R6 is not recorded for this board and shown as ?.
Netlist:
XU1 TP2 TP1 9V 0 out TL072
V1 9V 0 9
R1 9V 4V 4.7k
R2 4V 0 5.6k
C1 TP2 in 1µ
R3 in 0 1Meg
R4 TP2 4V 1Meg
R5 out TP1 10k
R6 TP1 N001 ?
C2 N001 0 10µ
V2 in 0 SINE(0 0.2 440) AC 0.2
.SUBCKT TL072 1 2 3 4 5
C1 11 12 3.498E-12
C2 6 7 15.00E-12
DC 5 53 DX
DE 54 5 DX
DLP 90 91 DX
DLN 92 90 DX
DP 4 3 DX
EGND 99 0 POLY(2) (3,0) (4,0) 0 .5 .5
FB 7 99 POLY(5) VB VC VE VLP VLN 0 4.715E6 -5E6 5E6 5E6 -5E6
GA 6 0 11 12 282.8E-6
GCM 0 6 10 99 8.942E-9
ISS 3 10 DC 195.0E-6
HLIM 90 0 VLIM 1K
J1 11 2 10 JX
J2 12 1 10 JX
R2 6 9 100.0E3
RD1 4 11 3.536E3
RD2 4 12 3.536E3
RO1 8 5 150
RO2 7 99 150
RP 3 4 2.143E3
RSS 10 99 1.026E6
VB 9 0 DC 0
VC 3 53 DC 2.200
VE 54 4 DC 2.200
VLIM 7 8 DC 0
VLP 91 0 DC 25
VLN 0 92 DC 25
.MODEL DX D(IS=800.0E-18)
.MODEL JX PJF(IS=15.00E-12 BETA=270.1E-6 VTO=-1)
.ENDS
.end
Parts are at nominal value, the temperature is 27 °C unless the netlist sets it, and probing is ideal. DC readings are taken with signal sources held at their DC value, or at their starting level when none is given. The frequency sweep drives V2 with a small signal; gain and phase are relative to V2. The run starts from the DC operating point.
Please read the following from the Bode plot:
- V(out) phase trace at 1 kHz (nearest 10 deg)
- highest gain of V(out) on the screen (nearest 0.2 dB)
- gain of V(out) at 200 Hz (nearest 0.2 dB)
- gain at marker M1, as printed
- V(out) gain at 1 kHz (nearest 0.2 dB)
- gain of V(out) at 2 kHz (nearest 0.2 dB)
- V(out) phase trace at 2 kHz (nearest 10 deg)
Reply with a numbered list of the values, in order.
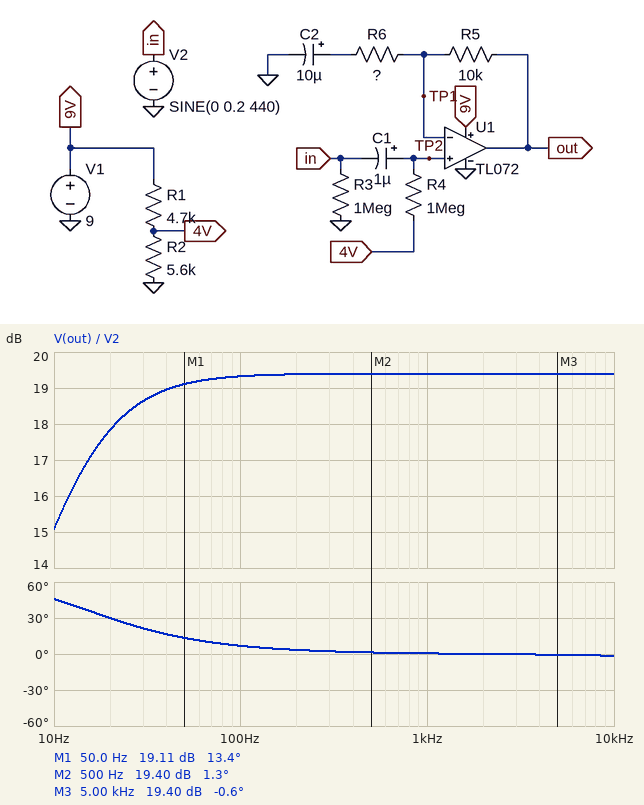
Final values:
1. 0 deg
2. 19.4 dB
3. 19.4 dB
4. 19.11 dB
5. 19.4 dB
6. 19.4 dB
7. 0 deg
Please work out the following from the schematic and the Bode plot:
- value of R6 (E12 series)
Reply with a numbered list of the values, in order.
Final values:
1. 1.2 kΩ
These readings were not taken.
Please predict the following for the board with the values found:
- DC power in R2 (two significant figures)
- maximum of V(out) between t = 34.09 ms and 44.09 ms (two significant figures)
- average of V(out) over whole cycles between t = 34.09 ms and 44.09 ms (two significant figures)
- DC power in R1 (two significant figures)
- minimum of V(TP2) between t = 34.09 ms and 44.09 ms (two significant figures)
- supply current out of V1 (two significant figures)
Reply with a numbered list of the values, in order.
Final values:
1. 4.3 mW
2. 6.8 V
3. 4.9 V
4. 3.6 mW
5. 4.7 V
6. 5.3 mA
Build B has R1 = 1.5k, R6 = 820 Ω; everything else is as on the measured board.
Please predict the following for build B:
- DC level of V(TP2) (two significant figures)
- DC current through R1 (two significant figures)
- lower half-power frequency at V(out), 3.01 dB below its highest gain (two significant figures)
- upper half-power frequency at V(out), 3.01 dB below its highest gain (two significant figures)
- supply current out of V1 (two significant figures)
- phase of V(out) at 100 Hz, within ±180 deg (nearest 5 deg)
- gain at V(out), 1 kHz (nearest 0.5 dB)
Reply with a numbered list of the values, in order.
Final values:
1. 7.1 V
2. 1.3 mA
3. 19 Hz
4. 270 kHz
5. 5.7 mA
6. 10 deg
7. 22.5 dB
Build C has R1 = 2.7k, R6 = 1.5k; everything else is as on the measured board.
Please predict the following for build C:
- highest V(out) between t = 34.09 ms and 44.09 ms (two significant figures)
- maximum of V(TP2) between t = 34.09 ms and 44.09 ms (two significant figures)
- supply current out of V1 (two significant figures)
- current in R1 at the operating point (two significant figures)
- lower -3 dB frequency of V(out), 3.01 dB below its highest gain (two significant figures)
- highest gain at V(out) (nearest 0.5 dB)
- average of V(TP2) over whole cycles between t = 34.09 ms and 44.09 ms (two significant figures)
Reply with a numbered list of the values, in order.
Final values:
1. 7.4 V
2. 6.3 V
3. 5.5 mA
4. 1.1 mA
5. 10 Hz
6. 17.5 dB
7. 6.1 V
